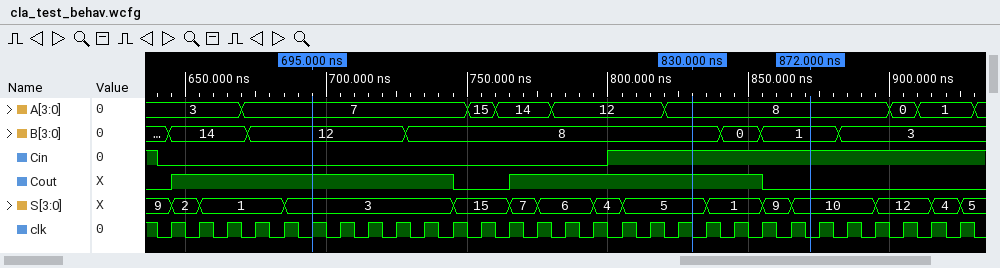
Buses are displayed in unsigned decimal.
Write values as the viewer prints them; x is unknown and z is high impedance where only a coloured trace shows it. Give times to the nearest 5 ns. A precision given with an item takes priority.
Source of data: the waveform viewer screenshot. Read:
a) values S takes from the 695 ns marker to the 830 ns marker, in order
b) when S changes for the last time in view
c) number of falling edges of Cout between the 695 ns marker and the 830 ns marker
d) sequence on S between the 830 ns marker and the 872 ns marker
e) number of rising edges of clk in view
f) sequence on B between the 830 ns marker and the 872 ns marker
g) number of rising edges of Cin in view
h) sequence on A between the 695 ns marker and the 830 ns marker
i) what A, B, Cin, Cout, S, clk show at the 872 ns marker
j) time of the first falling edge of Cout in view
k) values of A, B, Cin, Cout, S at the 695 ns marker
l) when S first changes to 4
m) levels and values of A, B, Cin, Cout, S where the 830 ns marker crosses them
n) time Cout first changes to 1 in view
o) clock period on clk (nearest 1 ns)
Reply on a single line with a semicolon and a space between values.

3, 15, 7, 6, 4, 5; 925 ns; 1; 5, 1, 9, 10; 29; 8, 0, 1; 1; 7, 15, 14, 12, 8; A=8, B=1, Cin=1, Cout=0, S=10, clk=0; 745 ns; A=7, B=12, Cin=0, Cout=1, S=3; 795 ns; A=8, B=8, Cin=1, Cout=1, S=5; 645 ns; 10 ns
